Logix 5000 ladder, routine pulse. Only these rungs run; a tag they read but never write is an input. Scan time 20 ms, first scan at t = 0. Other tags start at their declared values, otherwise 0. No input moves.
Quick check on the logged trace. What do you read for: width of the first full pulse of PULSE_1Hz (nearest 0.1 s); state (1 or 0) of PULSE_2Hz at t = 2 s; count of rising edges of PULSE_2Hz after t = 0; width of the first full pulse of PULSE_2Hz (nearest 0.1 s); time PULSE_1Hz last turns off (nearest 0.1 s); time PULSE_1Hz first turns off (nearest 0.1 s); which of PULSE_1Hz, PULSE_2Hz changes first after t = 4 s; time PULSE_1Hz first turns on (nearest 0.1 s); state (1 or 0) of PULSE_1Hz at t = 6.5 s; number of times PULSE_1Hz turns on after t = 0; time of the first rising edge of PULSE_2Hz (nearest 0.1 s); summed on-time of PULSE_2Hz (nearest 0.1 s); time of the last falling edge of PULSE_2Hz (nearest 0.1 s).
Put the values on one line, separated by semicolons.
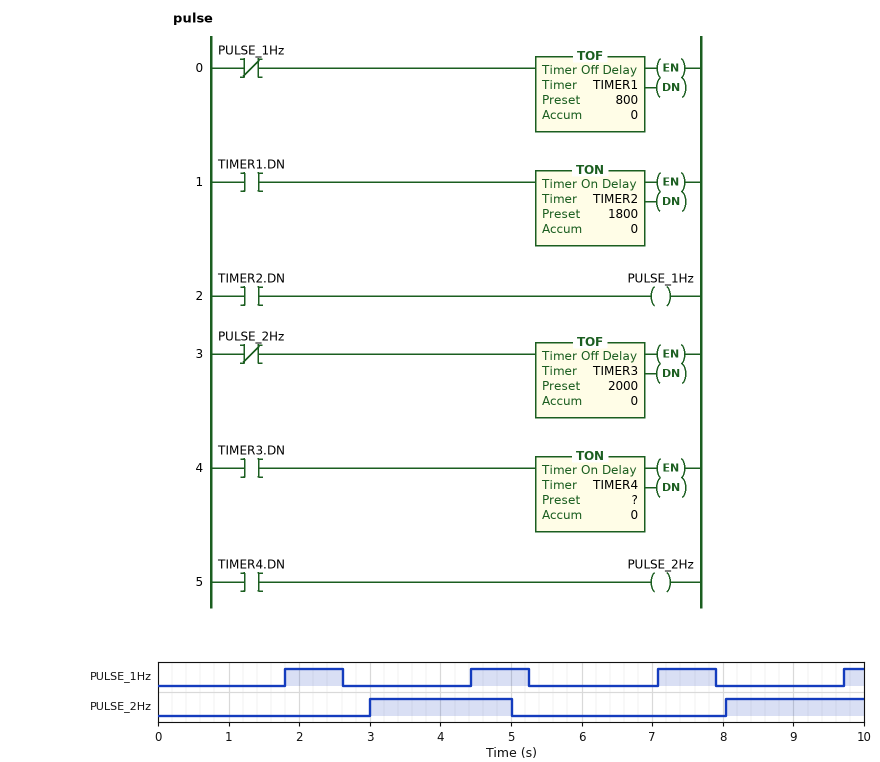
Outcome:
0.8 s; 0; 2; 2.0 s; 7.9 s; 2.6 s; PULSE_1Hz; 1.8 s; 0; 4; 3.0 s; 4.0 s; 5.0 s
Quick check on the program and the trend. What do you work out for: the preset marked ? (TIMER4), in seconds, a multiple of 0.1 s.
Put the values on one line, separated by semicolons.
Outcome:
3.0 s
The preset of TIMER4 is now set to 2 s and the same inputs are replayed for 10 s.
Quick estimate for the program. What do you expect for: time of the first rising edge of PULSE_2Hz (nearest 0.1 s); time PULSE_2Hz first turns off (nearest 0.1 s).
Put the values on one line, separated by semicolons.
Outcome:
2.0 s; 4.0 s
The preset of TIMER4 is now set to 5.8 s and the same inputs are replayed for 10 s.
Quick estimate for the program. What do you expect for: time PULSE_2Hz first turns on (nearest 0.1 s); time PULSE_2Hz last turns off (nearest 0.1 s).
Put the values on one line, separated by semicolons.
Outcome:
5.8 s; 7.8 s
